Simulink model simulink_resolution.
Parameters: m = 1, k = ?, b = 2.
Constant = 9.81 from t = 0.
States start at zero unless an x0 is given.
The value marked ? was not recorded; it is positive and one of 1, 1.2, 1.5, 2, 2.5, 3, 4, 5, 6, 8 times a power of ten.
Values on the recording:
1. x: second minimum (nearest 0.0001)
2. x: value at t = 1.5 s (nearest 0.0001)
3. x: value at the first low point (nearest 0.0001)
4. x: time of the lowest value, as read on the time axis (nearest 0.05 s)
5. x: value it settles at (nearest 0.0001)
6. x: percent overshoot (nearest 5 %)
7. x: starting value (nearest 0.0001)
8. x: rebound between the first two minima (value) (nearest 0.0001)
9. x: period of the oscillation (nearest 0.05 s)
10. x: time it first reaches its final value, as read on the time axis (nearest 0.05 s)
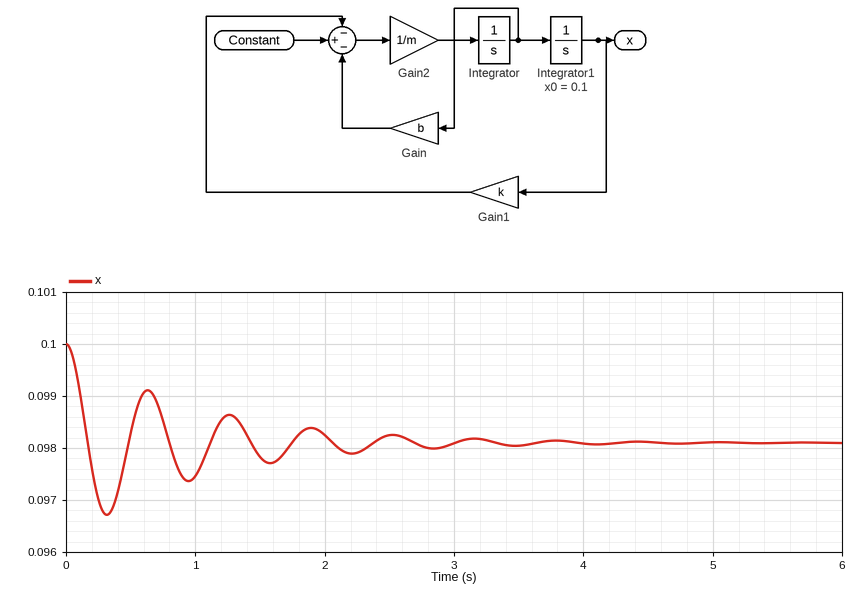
0.0974
0.0978
0.0967
0.30 s
0.0981
75 %
0.1000
0.0991
0.65 s
0.15 s
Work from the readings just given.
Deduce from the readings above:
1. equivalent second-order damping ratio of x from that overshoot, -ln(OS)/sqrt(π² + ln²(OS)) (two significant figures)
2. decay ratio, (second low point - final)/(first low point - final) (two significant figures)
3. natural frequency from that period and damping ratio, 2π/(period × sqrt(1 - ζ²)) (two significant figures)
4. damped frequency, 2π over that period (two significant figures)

0.091
0.50
9.7 rad/s
9.7 rad/s
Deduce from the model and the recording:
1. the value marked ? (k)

100
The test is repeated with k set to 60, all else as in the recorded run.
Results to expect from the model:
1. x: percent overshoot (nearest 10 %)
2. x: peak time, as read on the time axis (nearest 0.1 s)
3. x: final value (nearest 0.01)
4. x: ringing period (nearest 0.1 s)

70 %
0.4 s
0.16
0.8 s
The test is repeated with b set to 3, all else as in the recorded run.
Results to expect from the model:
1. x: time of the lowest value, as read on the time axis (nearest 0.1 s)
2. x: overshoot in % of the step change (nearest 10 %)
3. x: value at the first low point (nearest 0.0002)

0.3 s
60 %
0.0970
